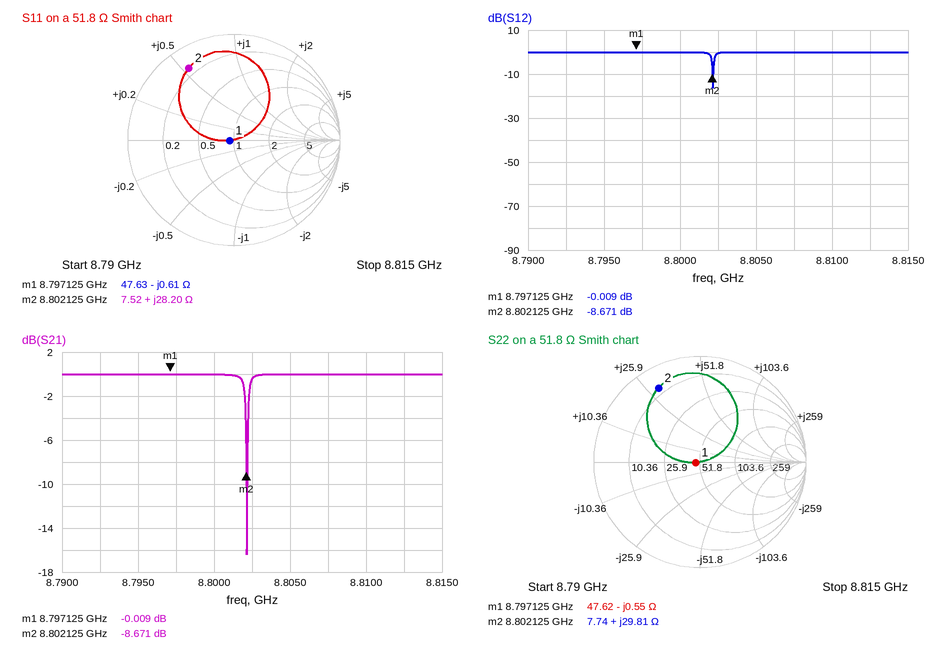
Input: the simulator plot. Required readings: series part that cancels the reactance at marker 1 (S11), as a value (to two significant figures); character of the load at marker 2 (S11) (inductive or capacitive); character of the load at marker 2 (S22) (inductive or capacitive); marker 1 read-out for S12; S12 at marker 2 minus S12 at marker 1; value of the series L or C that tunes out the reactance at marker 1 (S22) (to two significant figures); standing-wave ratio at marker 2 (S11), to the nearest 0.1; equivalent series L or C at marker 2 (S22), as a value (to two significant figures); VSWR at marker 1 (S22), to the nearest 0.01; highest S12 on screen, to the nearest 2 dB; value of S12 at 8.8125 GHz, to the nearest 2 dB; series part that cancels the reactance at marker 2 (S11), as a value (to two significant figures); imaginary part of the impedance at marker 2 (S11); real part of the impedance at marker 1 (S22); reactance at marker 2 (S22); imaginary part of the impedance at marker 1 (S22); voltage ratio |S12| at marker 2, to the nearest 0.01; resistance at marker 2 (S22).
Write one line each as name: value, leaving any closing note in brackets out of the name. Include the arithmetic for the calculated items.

series part that cancels the reactance at marker 1 (S11), as a value: L = 0.61 Ω/(2π × 8.797125 GHz) ≈ 11 pH
character of the load at marker 2 (S11): inductive
character of the load at marker 2 (S22): inductive
marker 1 read-out for S12: -0.009 dB
S12 at marker 2 minus S12 at marker 1: -8.671 − (-0.009) = -8.662 dB
value of the series L or C that tunes out the reactance at marker 1 (S22): L = 0.55 Ω/(2π × 8.797125 GHz) ≈ 10 pH
standing-wave ratio at marker 2 (S11), to the nearest 0.1: 9.0
equivalent series L or C at marker 2 (S22), as a value: L = 29.81 Ω/(2π × 8.802125 GHz) ≈ 539 pH, so 540 pH to two significant figures
VSWR at marker 1 (S22), to the nearest 0.01: 1.09
highest S12 on screen, to the nearest 2 dB: 0 dB
value of S12 at 8.8125 GHz, to the nearest 2 dB: 0 dB
series part that cancels the reactance at marker 2 (S11), as a value: C = 1/(2π × 8.802125 GHz × 28.2 Ω) ≈ 641 fF, so 640 fF to two significant figures
imaginary part of the impedance at marker 2: +28.20 Ω
real part of the impedance at marker 1: 47.62 Ω
reactance at marker 2: +29.81 Ω
imaginary part of the impedance at marker 1: -0.55 Ω
voltage ratio |S12| at marker 2, to the nearest 0.01: 10^(-8.671/20) ≈ 0.37
resistance at marker 2: 7.74 Ω
